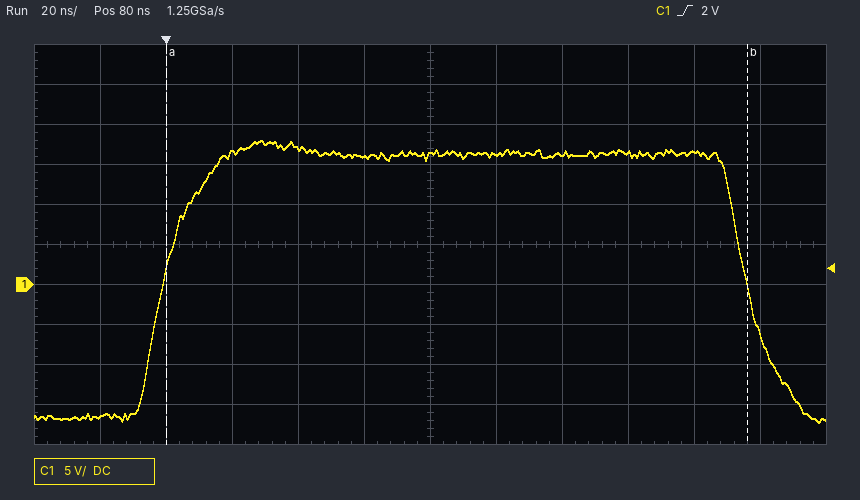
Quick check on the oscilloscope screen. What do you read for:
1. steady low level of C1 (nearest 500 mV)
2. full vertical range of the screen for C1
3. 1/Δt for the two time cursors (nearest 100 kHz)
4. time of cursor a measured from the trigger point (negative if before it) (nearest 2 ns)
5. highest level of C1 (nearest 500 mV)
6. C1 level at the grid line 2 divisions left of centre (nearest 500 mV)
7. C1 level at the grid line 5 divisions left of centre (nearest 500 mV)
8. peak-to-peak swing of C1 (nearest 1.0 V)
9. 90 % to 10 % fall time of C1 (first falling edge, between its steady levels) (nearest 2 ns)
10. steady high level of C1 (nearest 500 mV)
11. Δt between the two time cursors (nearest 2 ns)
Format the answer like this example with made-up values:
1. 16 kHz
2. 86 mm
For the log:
1. -16.5 V
2. 50 V
3. 5.7 MHz
4. 0 ns
5. 18.0 V
6. 17.0 V
7. -16.5 V
8. 35.0 V
9. 20 ns
10. 16.5 V
11. 176 ns
